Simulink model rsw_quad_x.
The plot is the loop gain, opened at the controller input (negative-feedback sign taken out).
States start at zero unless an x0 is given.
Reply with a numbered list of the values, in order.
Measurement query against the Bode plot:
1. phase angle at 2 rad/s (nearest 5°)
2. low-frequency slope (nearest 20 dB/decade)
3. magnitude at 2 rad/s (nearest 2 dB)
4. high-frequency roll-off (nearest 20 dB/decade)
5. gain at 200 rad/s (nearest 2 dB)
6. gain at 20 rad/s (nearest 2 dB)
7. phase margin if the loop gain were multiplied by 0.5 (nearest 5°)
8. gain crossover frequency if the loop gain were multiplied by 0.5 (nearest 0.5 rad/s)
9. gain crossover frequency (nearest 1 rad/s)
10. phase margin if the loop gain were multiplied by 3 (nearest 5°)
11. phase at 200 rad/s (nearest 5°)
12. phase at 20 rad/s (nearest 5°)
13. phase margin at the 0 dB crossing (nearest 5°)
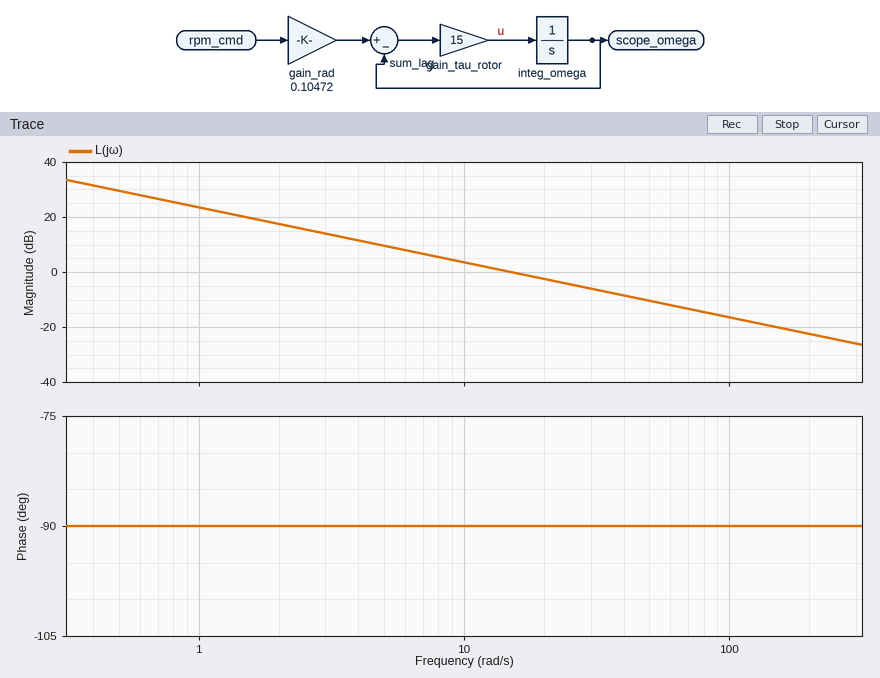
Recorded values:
1. -90°
2. -20 dB/decade
3. 18 dB
4. -20 dB/decade
5. -22 dB
6. -2 dB
7. 90°
8. 7.5 rad/s
9. 15 rad/s
10. 90°
11. -90°
12. -90°
13. 90°
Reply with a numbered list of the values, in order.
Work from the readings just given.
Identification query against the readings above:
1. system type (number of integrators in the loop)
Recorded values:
1. 1
